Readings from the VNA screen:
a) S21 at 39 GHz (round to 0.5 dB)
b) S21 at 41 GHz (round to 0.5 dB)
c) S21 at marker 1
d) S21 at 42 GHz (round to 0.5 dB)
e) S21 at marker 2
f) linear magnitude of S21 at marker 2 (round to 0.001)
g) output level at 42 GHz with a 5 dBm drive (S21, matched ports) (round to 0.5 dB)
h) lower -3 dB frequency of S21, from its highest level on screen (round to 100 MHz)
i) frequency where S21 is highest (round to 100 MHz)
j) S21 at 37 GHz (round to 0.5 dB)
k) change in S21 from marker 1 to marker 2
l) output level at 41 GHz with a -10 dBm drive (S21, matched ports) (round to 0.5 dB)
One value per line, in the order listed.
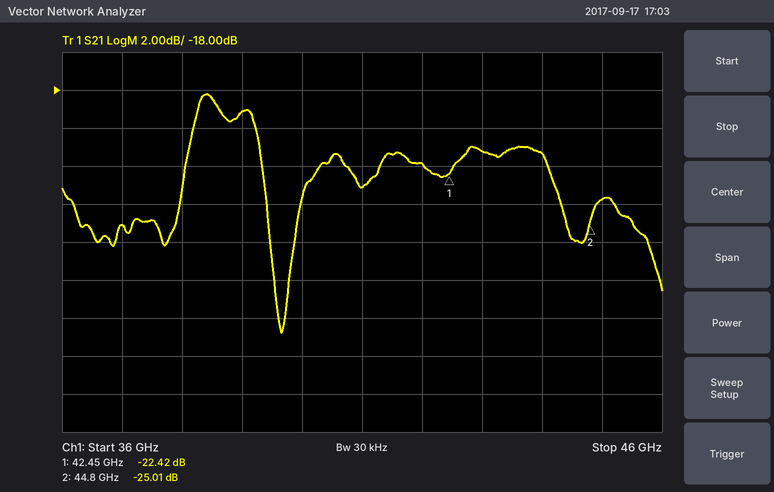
-19.0 dB
-23.0 dB
-22.42 dB
-22.0 dB
-25.01 dB
0.056
-17.0 dBm
38.1 GHz
38.4 GHz
-25.0 dB
-2.59 dB
-33.0 dBm
